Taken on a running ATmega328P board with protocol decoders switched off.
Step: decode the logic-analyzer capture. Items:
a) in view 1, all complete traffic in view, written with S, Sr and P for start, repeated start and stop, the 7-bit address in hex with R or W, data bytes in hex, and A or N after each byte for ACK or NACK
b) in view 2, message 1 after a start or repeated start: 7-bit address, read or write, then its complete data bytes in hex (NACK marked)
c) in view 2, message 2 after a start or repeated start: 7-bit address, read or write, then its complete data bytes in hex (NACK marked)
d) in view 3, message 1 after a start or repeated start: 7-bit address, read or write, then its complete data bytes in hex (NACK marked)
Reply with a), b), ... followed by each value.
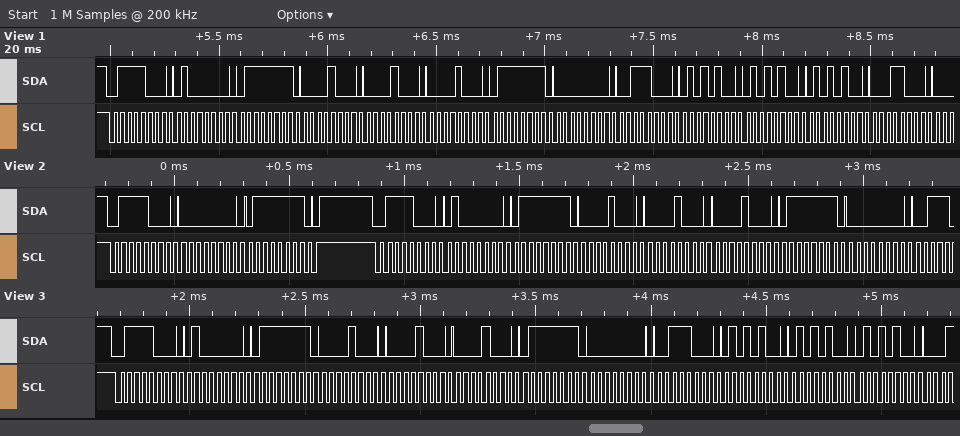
a) S 3CW A 40 A 7F A 08 A 08 A 08 A 7F A 00 A 38 A 54 A 54 A 54 A 18 A
b) 0x3C write: 00 7F
c) 0x3C write: 40 7F 08 08 08 7F 00
d) 0x3C write: 40 7F 08 08 08 7F 00 38 54 54 54
